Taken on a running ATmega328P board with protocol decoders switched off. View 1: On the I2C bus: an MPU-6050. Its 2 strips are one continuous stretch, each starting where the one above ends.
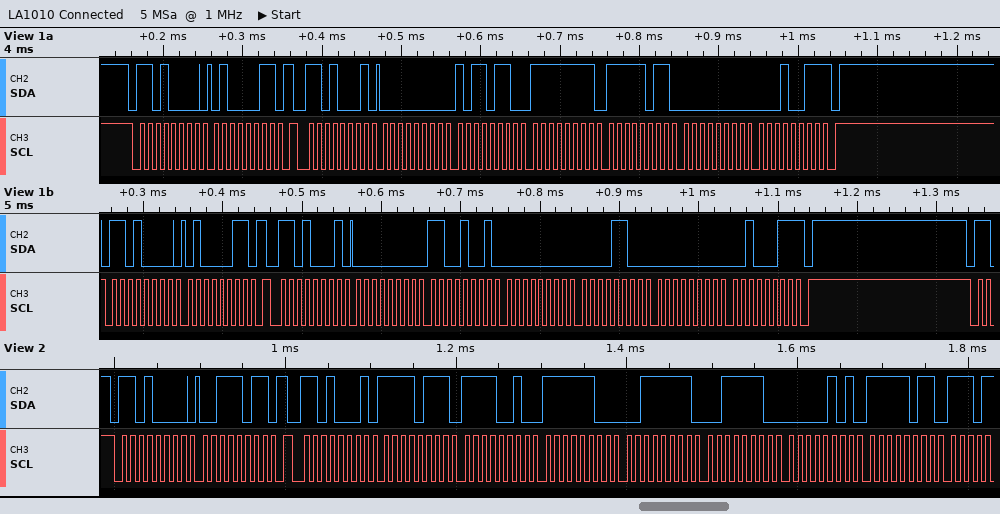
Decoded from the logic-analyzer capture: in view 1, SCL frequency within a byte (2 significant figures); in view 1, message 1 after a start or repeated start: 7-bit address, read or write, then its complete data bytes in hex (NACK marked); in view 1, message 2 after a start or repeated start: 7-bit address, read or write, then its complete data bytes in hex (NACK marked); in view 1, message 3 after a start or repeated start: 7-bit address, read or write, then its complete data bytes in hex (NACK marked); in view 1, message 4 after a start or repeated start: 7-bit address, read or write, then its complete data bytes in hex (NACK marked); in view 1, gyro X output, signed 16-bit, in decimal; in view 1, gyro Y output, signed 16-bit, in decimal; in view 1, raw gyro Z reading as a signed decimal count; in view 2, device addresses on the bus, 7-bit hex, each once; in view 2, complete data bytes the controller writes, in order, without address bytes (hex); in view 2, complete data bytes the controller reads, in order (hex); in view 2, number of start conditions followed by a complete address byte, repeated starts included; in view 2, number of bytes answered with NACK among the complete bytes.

100 kHz
0x68 write: 43
0x68 read: 00 B6 FF FB 00 13 NACK
0x68 write: 43
0x68 read: 00 C9 00 0C 00 23 NACK
182
-5
19
0x68
3B
F7 F2 FC 3F 3E 05 FB
2
0
